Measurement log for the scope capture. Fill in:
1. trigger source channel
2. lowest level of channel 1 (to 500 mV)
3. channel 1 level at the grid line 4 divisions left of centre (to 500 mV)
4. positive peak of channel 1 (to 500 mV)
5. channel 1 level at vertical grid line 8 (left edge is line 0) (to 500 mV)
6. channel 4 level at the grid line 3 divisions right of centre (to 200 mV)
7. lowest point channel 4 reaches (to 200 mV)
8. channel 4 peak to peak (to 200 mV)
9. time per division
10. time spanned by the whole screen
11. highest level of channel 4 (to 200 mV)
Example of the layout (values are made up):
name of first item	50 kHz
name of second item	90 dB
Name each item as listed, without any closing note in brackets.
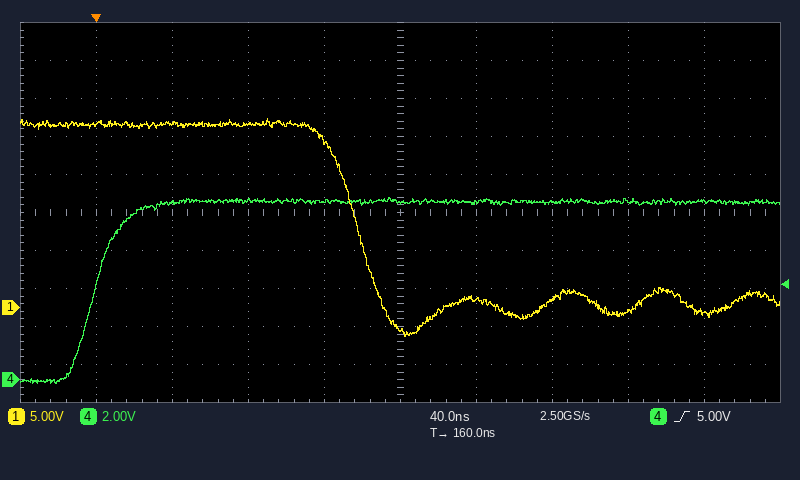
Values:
trigger source channel	channel 4
lowest level of channel 1	-4.0 V
channel 1 level at the grid line 4 divisions left of centre	24.0 V
positive peak of channel 1	25.0 V
channel 1 level at vertical grid line 8 (left edge is line 0)	-500 mV
channel 4 level at the grid line 3 divisions right of centre	9.4 V
lowest point channel 4 reaches	-200 mV
channel 4 peak to peak	9.8 V
time per division	40 ns
time spanned by the whole screen	400 ns
highest level of channel 4	9.6 V
